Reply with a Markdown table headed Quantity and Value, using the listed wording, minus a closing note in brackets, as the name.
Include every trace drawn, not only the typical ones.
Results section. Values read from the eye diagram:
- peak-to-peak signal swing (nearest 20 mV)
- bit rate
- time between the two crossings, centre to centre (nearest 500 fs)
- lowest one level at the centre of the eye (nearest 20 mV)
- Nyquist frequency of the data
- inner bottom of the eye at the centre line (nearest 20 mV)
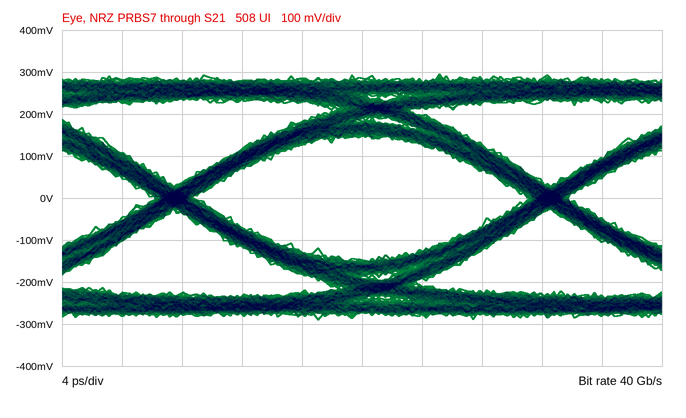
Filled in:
| Quantity | Value |
|---|---|
| peak-to-peak signal swing | 580 mV |
| bit rate | 40 Gb/s |
| time between the two crossings, centre to centre | 25.0 ps |
| lowest one level at the centre of the eye | 140 mV |
| Nyquist frequency of the data | 20 GHz |
| inner bottom of the eye at the centre line | -140 mV |
